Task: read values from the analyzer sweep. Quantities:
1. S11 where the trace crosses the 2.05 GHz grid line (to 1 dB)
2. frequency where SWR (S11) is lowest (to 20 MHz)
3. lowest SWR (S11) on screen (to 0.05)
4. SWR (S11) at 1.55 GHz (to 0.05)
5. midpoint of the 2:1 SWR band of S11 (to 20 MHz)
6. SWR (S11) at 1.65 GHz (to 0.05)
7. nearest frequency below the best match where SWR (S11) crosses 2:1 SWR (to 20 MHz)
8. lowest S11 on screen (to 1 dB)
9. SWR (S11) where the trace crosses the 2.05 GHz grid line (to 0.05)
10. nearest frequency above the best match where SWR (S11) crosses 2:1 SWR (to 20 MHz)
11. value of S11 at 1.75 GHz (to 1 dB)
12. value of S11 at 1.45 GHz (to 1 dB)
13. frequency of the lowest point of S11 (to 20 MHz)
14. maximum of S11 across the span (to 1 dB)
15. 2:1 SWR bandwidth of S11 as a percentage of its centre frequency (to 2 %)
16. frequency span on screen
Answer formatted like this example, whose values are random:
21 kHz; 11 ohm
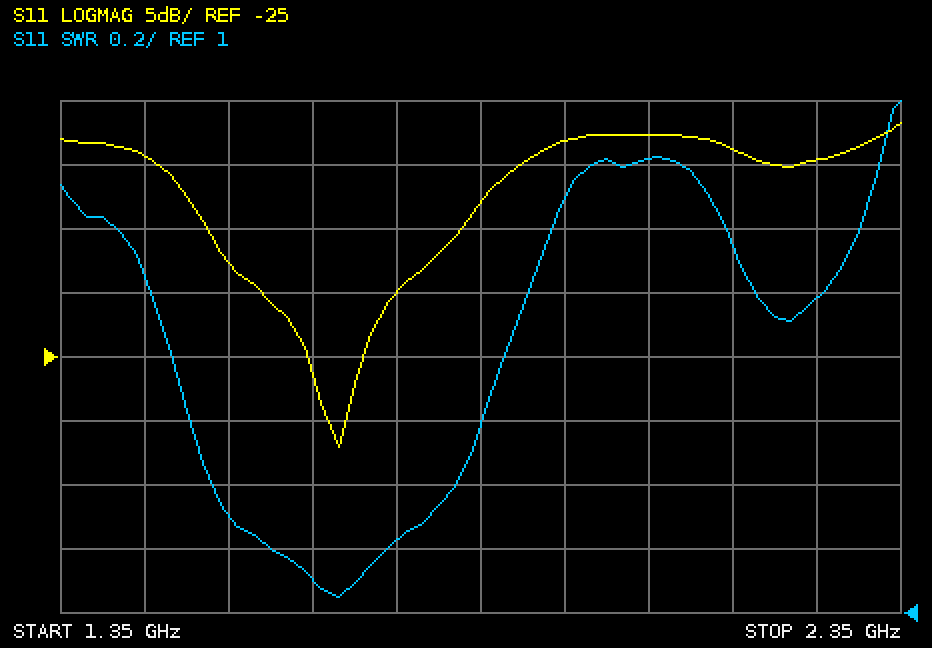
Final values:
-8 dB; 1.68 GHz; 1.05; 1.30; 1.68 GHz; 1.10; 1.46 GHz; -32 dB; 2.40; 1.90 GHz; -20 dB; -9 dB; 1.68 GHz; -7 dB; 26 %; 1 GHz
